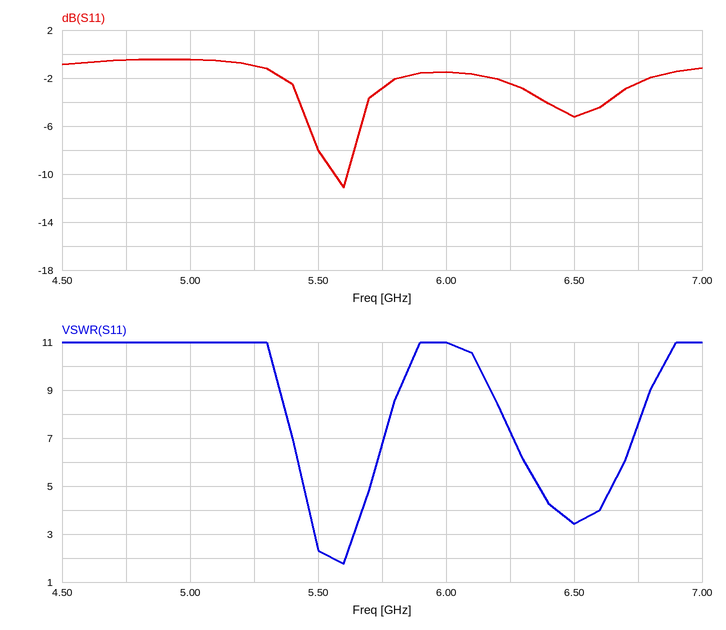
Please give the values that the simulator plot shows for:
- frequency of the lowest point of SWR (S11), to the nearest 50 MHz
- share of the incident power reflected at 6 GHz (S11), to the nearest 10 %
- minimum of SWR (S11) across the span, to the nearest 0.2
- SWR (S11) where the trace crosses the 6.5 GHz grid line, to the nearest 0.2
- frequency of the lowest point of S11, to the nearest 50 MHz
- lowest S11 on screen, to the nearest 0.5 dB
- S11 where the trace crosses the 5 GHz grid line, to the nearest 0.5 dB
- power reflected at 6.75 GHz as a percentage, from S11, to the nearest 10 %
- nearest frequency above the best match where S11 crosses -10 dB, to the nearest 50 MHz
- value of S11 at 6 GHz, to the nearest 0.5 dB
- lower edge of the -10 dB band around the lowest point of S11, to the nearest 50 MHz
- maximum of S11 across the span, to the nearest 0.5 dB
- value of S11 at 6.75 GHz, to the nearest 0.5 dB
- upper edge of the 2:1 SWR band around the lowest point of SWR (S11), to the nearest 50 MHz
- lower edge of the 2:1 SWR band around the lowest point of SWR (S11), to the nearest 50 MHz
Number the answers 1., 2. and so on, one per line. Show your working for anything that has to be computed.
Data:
1. 5.60 GHz
2. 10^(-1.5/10) ≈ 70.8 %, so 70 % to the nearest 10 %
3. 1.8
4. 3.4
5. 5.60 GHz
6. -11.0 dB
7. -0.5 dB
8. 10^(-2.5/10) ≈ 56.2 %, so 60 % to the nearest 10 %
9. 5.60 GHz
10. -1.5 dB
11. 5.55 GHz
12. -0.5 dB
13. -2.5 dB
14. 5.60 GHz
15. 5.55 GHz
